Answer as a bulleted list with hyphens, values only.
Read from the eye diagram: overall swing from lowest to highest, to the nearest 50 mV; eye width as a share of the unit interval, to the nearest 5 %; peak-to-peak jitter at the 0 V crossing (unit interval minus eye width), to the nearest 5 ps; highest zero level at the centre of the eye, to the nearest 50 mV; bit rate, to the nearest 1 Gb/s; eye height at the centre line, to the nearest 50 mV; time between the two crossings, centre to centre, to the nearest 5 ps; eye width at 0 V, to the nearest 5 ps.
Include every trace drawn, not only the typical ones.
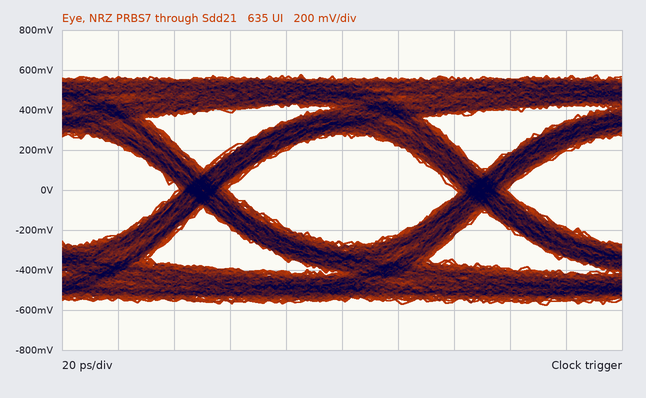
- 1.15 V
- 80 %
- 20 ps
- -250 mV
- 10 Gb/s
- 550 mV
- 100 ps
- 80 ps
